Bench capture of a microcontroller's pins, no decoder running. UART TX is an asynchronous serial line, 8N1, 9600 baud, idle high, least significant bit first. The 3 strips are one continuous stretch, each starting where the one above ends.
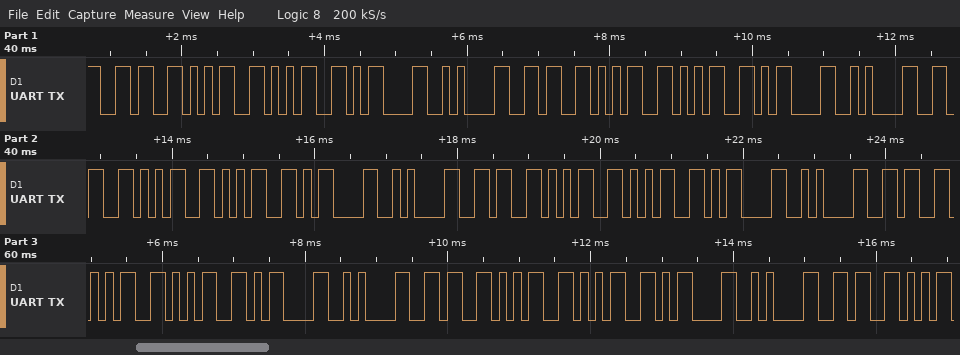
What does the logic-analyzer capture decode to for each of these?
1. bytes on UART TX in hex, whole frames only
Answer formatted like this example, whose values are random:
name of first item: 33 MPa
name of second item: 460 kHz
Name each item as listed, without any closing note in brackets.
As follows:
bytes on UART TX in hex, whole frames only: 36 35 35 0D 0A 36 35 35 0D 0A 36 35 35 0D 0A 36 35 35 0D 0A 36 35 35 0D 0A 36 35 35 0D 0A 36
